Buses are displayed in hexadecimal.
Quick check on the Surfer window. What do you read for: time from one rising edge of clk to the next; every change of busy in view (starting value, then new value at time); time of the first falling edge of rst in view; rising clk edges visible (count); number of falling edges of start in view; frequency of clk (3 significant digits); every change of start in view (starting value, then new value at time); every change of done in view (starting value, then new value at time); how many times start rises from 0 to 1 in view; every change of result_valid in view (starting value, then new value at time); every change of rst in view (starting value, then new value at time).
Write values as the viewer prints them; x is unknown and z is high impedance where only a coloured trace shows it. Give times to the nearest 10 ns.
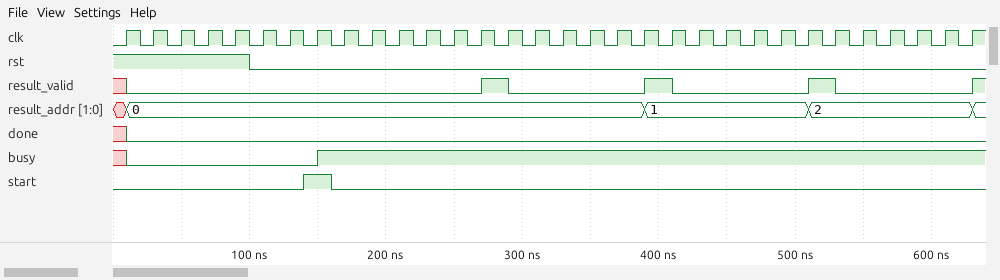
20 ns
x, 0 at 10 ns, 1 at 150 ns
100 ns
32
1
50.0 MHz
0, 1 at 140 ns, 0 at 160 ns
x, 0 at 10 ns
1
x, 0 at 10 ns, 1 at 270 ns, 0 at 290 ns, 1 at 390 ns, 0 at 410 ns, 1 at 510 ns, 0 at 530 ns, 1 at 630 ns
1, 0 at 100 ns
